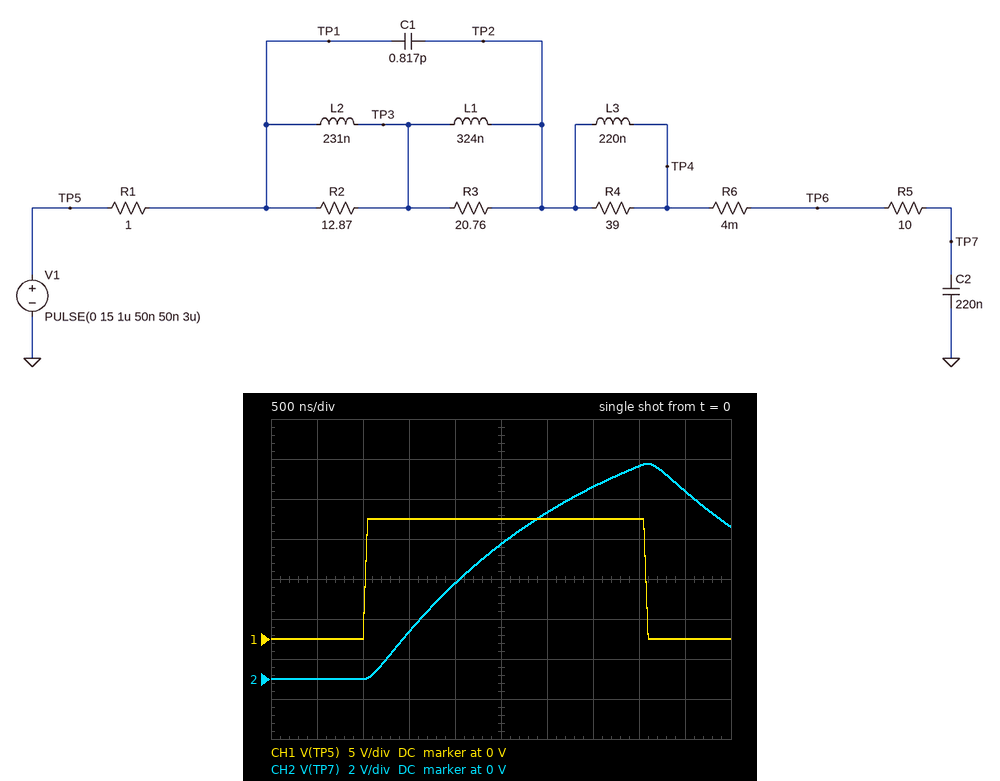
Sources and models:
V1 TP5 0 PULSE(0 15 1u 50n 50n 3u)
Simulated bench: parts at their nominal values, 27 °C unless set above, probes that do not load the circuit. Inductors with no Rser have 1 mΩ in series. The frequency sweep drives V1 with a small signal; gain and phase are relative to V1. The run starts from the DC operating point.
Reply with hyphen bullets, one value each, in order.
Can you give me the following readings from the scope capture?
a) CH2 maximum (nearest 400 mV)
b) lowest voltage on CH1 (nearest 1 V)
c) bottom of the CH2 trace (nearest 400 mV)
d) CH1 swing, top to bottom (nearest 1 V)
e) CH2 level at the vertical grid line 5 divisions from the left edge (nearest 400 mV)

- 10.8 V
- 0 V
- 0 V
- 15 V
- 6.8 V
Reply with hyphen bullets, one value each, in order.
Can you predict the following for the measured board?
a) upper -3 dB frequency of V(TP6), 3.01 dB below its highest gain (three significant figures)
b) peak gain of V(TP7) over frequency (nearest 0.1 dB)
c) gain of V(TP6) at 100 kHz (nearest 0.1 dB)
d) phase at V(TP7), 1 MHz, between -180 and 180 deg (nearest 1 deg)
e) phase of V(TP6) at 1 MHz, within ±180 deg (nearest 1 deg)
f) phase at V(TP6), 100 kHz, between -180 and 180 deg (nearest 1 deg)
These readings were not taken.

- 1.64 MHz
- 0 dB
- -0.4 dB
- -110 deg
- -24 deg
- -4 deg
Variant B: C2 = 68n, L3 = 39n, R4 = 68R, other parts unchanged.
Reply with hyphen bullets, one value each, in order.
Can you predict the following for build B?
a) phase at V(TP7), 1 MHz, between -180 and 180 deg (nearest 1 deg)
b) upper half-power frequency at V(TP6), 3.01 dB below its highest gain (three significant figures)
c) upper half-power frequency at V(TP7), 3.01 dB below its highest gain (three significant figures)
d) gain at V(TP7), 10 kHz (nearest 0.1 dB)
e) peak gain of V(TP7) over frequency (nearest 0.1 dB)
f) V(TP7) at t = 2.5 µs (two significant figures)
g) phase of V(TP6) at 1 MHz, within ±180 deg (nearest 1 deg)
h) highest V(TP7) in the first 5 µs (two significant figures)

- -97 deg
- 2.15 MHz
- 229 kHz
- 0 dB
- 0 dB
- 13 V
- -20 deg
- 15 V
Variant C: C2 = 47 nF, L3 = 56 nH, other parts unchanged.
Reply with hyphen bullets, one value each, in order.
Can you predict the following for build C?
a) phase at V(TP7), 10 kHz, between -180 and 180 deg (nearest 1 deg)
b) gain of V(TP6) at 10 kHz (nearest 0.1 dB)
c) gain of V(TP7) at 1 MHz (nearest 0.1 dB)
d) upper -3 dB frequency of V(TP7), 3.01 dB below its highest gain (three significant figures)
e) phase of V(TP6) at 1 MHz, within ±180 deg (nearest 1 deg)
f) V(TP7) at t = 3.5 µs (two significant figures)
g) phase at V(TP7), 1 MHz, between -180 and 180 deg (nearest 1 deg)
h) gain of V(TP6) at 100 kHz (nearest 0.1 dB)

- -2 deg
- 0 dB
- -10.5 dB
- 342 kHz
- -21 deg
- 15 V
- -92 deg
- 0 dB
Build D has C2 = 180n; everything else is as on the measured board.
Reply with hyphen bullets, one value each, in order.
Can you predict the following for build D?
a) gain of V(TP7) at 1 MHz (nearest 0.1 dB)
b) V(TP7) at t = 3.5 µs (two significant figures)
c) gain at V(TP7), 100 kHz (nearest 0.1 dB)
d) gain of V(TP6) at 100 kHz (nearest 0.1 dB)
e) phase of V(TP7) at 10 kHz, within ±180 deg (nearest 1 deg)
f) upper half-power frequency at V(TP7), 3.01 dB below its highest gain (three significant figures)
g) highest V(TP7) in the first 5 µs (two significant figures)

- -22.7 dB
- 11 V
- -3.9 dB
- -0.3 dB
- -7 deg
- 83.3 kHz
- 12 V
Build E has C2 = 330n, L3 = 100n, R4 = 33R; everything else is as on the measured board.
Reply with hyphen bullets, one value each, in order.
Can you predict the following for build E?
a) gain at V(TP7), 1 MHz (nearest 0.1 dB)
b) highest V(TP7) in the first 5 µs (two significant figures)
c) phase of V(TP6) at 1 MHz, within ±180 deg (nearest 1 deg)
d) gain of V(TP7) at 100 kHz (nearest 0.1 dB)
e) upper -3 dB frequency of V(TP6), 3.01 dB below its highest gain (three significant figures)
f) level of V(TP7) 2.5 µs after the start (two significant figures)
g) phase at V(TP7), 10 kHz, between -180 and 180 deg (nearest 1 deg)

- -27.9 dB
- 8.5 V
- -20 deg
- -7.8 dB
- 1.84 MHz
- 4.9 V
- -13 deg
